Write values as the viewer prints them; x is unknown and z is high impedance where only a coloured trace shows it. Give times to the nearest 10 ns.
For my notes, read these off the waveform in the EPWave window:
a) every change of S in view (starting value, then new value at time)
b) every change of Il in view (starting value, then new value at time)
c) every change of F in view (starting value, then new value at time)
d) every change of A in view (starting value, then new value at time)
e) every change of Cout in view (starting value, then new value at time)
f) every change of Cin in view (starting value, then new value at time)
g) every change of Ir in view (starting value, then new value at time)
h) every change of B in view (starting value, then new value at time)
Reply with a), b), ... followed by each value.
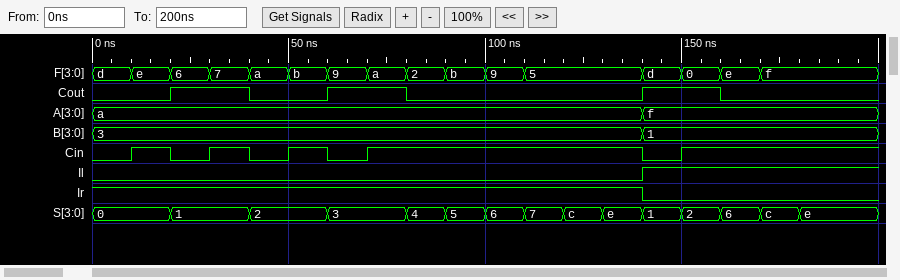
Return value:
a) 0, 1 at 20 ns, 2 at 40 ns, 3 at 60 ns, 4 at 80 ns, 5 at 90 ns, 6 at 100 ns, 7 at 110 ns, c at 120 ns, e at 130 ns, 1 at 140 ns, 2 at 150 ns, 6 at 160 ns, c at 170 ns, e at 180 ns
b) 0, 1 at 140 ns
c) d, e at 10 ns, 6 at 20 ns, 7 at 30 ns, a at 40 ns, b at 50 ns, 9 at 60 ns, a at 70 ns, 2 at 80 ns, b at 90 ns, 9 at 100 ns, 5 at 110 ns, d at 140 ns, 0 at 150 ns, e at 160 ns, f at 170 ns
d) a, f at 140 ns
e) 0, 1 at 20 ns, 0 at 40 ns, 1 at 60 ns, 0 at 80 ns, 1 at 140 ns, 0 at 160 ns
f) 0, 1 at 10 ns, 0 at 20 ns, 1 at 30 ns, 0 at 40 ns, 1 at 50 ns, 0 at 60 ns, 1 at 70 ns, 0 at 140 ns, 1 at 150 ns
g) 1, 0 at 140 ns
h) 3, 1 at 140 ns
